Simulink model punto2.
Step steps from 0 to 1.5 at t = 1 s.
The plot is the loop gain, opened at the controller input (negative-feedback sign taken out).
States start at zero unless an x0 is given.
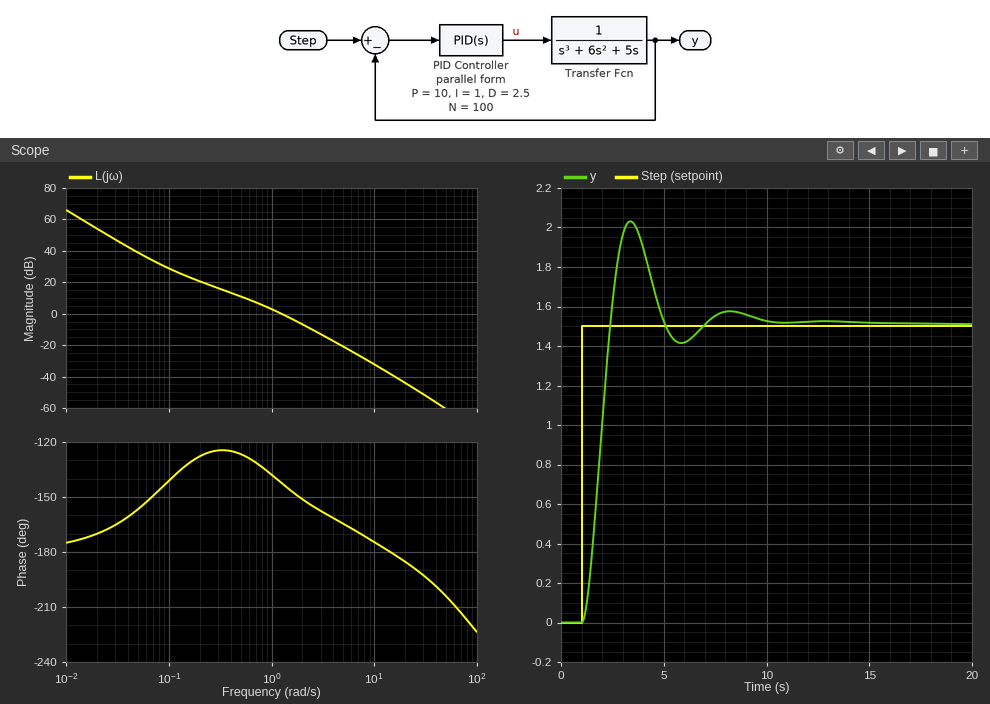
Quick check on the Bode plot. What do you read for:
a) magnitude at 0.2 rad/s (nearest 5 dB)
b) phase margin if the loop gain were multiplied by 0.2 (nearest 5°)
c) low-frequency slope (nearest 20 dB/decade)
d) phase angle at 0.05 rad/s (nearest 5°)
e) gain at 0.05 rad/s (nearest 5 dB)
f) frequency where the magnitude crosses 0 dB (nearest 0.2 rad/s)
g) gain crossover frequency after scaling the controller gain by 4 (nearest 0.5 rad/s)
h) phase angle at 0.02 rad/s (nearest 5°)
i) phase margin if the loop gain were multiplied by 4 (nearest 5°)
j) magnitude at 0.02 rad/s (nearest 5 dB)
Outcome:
20 dB
55°
-40 dB/decade
-155°
40 dB
1.2 rad/s
3.0 rad/s
-170°
25°
55 dB
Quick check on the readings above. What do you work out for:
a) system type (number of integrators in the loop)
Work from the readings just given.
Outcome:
2
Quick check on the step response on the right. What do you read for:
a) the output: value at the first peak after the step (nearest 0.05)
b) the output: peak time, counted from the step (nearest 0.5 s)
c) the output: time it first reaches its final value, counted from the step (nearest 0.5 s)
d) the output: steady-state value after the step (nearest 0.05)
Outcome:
2.05
2.5 s
1.5 s
1.50
